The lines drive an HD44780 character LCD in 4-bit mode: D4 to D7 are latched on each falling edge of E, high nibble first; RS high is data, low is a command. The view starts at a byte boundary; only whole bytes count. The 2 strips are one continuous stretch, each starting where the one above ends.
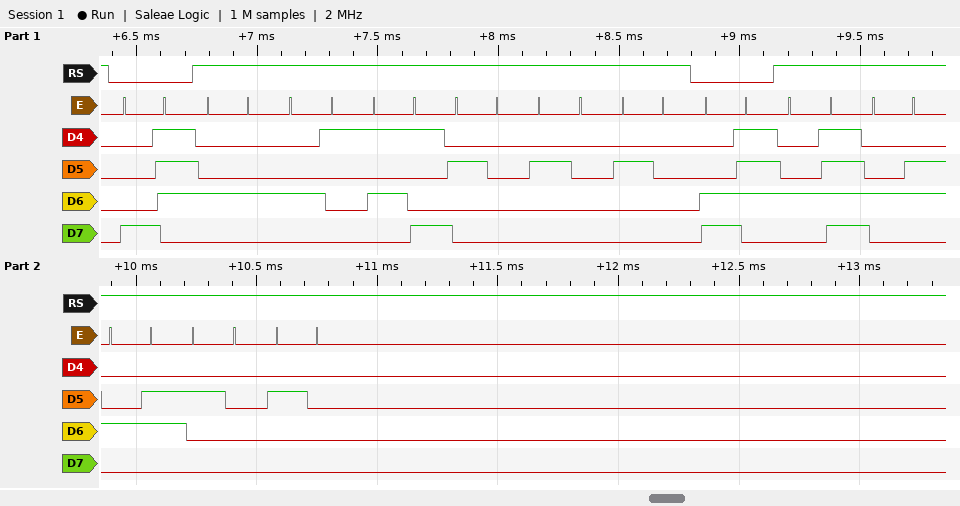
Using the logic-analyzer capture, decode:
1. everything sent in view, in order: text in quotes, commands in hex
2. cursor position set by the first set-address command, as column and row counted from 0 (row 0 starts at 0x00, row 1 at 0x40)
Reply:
0x87 "DAY   " 0xC7 "OFF  "
column 7, row 0
